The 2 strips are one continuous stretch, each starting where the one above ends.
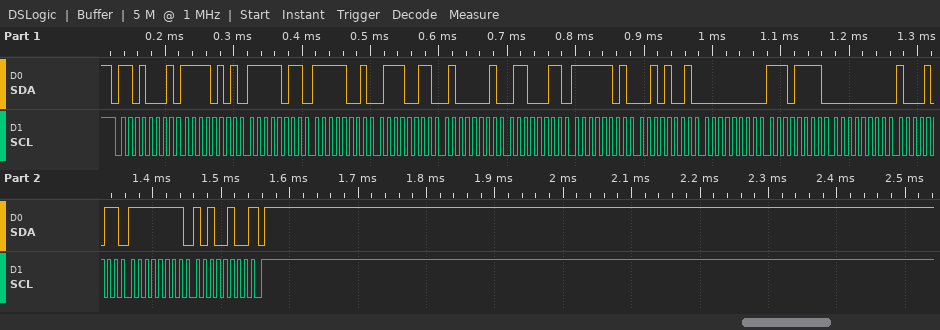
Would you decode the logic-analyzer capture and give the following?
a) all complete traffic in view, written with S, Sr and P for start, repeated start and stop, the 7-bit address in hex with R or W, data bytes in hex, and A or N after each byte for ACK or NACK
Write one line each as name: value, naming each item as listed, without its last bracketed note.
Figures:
all complete traffic in view, written with S, Sr and P for start, repeated start and stop, the 7-bit address in hex with R or W, data bytes in hex, and A or N after each byte for ACK or NACK: S 68R A F5 A FB A F9 A 73 A 41 A 63 A FD A 29 A 00 A EF A 00 A 8B A FF A A4 N P
